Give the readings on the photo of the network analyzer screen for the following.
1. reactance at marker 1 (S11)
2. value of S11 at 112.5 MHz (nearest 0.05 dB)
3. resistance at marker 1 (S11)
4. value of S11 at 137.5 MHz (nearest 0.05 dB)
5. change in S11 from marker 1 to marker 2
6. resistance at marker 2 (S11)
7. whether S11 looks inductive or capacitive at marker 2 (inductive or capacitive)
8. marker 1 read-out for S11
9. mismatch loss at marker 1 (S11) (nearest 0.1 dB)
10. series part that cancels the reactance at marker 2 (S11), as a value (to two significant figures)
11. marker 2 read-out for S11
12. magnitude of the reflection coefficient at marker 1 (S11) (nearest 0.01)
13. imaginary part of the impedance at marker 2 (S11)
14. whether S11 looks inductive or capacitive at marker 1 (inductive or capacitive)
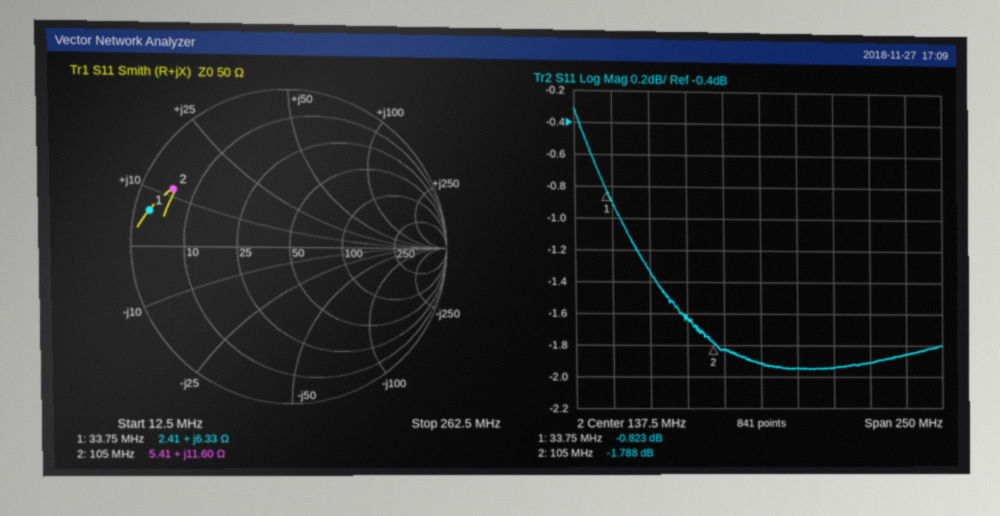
+6.33 Ω
-1.85 dB
2.41 Ω
-1.90 dB
-0.965 dB
5.41 Ω
inductive
-0.823 dB
7.6 dB
130 pF
-1.788 dB
0.91
+11.60 Ω
inductive
